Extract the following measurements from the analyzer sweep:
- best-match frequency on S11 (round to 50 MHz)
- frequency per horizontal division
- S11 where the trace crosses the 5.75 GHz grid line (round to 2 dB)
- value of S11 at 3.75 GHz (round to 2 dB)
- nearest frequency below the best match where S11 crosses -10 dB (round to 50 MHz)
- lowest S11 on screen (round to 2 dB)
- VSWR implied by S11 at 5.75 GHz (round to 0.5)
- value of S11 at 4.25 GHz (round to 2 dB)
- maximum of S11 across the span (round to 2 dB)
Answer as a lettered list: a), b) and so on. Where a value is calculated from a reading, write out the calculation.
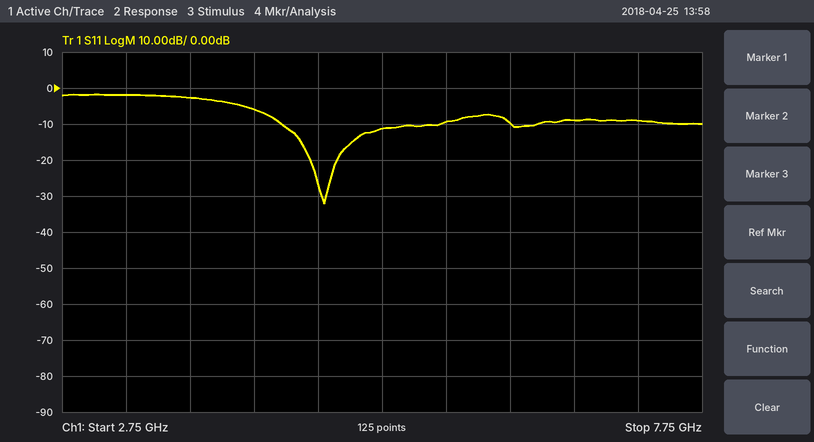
a) 4.80 GHz
b) 500 MHz
c) -10 dB
d) -2 dB
e) 4.45 GHz
f) -32 dB
g) |Γ| = 10^(-10/20) = 0.3162; VSWR = (1 + 0.3162)/(1 − 0.3162) ≈ 1.92, so 2.0 to the nearest 0.5
h) -6 dB
i) -2 dB
